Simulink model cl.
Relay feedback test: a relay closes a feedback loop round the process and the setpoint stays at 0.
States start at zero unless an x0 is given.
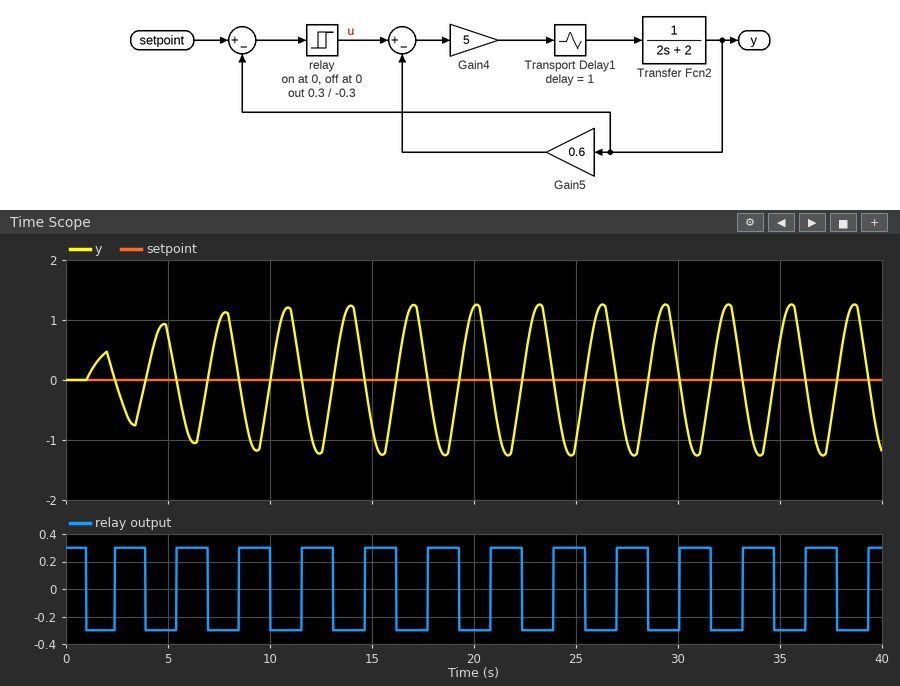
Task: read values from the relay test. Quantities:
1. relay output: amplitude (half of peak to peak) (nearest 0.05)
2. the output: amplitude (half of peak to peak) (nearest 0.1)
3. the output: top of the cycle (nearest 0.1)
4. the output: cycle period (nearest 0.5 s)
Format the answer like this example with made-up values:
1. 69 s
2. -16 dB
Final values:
1. 0.30
2. 1.3
3. 1.3
4. 3.0 s
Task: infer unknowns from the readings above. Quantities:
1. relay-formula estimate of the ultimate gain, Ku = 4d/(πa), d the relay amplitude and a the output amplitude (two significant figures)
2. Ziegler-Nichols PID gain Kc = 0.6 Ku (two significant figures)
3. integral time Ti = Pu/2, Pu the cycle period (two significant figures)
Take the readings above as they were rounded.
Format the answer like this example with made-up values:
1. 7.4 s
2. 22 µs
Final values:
1. 0.29
2. 0.17
3. 1.5 s
